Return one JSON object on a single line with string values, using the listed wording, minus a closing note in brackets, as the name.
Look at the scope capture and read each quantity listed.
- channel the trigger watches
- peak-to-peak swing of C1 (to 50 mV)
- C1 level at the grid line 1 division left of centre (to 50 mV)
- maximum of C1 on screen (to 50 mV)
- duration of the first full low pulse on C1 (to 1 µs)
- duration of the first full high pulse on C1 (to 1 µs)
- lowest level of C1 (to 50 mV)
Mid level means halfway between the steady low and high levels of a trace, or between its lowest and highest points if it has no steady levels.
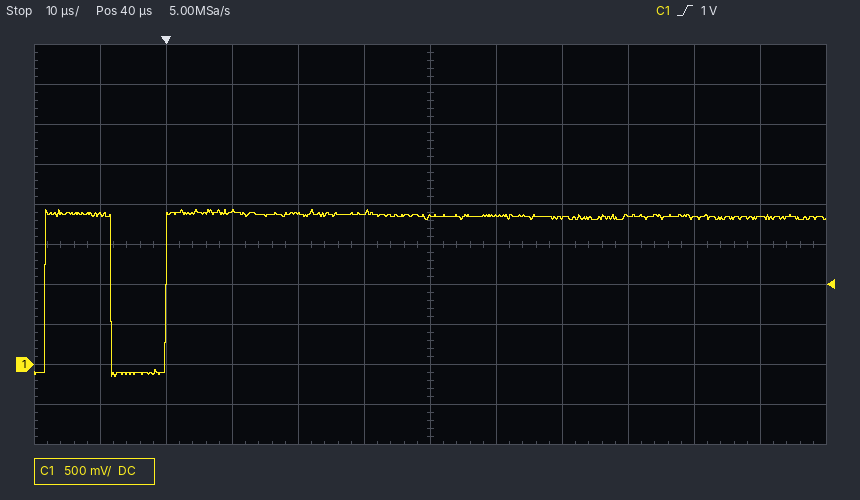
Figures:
{"channel the trigger watches": "C1", "peak-to-peak swing of C1": "2.10 V", "C1 level at the grid line 1 division left of centre": "1.90 V", "maximum of C1 on screen": "1.95 V", "duration of the first full low pulse on C1": "8 µs", "duration of the first full high pulse on C1": "10 µs", "lowest level of C1": "-150 mV"}
